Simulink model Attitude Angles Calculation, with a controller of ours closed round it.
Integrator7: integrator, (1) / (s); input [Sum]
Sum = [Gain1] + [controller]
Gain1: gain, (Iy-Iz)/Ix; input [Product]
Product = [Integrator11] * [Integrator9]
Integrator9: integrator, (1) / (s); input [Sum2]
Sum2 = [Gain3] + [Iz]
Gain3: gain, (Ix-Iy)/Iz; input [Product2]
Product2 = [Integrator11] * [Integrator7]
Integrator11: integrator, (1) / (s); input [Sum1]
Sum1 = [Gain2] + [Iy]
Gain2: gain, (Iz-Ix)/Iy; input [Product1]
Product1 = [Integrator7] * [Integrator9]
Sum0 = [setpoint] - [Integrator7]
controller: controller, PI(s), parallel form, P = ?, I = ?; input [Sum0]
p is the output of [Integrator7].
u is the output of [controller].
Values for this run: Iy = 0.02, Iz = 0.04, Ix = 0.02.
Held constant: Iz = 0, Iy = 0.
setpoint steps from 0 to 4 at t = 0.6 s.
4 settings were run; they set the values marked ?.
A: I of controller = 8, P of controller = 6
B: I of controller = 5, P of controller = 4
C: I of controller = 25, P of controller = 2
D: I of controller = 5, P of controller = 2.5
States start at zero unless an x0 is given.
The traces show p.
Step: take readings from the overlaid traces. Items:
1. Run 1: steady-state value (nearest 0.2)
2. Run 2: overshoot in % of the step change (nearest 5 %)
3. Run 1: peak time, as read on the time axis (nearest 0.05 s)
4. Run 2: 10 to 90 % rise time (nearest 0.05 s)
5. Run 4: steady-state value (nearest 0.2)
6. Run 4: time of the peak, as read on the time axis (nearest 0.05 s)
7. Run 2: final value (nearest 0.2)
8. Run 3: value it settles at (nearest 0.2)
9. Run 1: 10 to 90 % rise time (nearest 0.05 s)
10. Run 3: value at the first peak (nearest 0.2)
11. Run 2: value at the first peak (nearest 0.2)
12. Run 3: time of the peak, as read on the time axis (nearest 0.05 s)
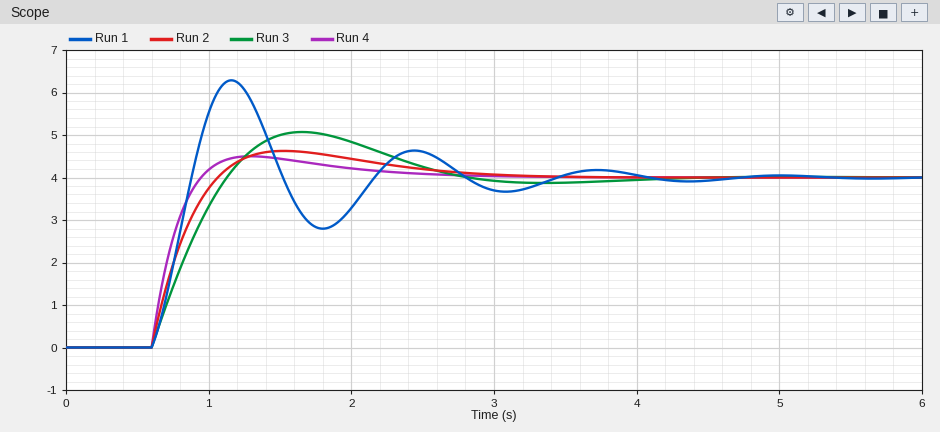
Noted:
4.0
15 %
1.15 s
0.35 s
4.0
1.30 s
4.0
4.0
0.20 s
5.0
4.6
1.65 s
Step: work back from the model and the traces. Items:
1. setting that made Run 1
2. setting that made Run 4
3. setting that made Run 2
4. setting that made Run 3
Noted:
C
A
B
D
